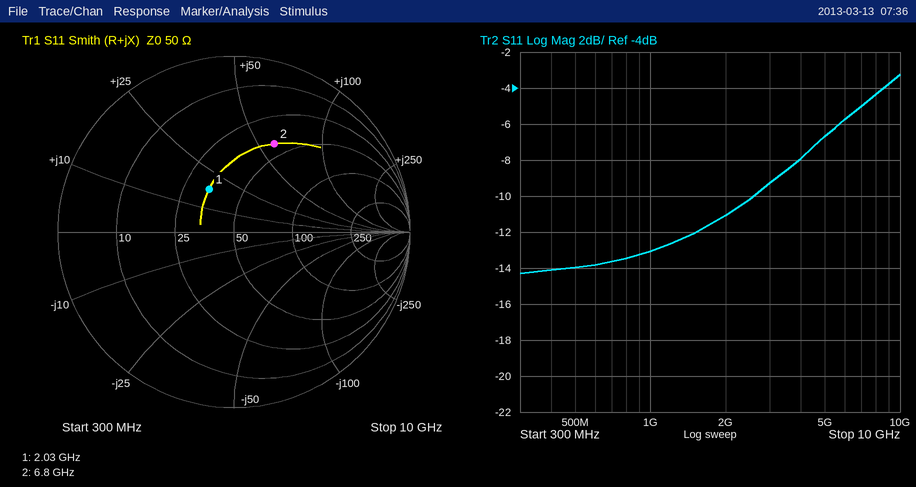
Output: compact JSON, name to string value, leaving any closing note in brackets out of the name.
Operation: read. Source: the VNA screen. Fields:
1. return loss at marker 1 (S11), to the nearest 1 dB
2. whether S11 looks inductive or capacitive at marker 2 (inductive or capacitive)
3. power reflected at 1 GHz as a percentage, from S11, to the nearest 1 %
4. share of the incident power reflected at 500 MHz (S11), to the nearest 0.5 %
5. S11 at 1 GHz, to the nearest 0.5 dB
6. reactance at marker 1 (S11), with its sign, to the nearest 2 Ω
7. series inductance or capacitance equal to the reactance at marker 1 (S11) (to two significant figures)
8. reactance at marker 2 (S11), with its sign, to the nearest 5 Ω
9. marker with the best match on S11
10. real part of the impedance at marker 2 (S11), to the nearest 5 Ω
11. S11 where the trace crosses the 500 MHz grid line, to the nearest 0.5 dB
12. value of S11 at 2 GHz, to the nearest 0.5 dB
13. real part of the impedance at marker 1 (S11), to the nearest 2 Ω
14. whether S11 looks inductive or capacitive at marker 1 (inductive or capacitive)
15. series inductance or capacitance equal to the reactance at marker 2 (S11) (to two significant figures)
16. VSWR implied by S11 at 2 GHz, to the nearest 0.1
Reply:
{"return loss at marker 1 (S11), to the nearest 1 dB": "11 dB", "whether S11 looks inductive or capacitive at marker 2": "inductive", "power reflected at 1 GHz as a percentage, from S11, to the nearest 1 %": "5 %", "share of the incident power reflected at 500 MHz (S11), to the nearest 0.5 %": "4.0 %", "S11 at 1 GHz, to the nearest 0.5 dB": "-13.0 dB", "reactance at marker 1 (S11), with its sign, to the nearest 2 Ω": "+18 Ω", "series inductance or capacitance equal to the reactance at marker 1 (S11)": "1.4 nH", "reactance at marker 2 (S11), with its sign, to the nearest 5 Ω": "+60 Ω", "marker with the best match on S11": "marker 1", "real part of the impedance at marker 2 (S11), to the nearest 5 Ω": "40 Ω", "S11 where the trace crosses the 500 MHz grid line, to the nearest 0.5 dB": "-14.0 dB", "value of S11 at 2 GHz, to the nearest 0.5 dB": "-11.0 dB", "real part of the impedance at marker 1 (S11), to the nearest 2 Ω": "34 Ω", "whether S11 looks inductive or capacitive at marker 1": "inductive", "series inductance or capacitance equal to the reactance at marker 2 (S11)": "1.4 nH", "VSWR implied by S11 at 2 GHz, to the nearest 0.1": "1.8"}
